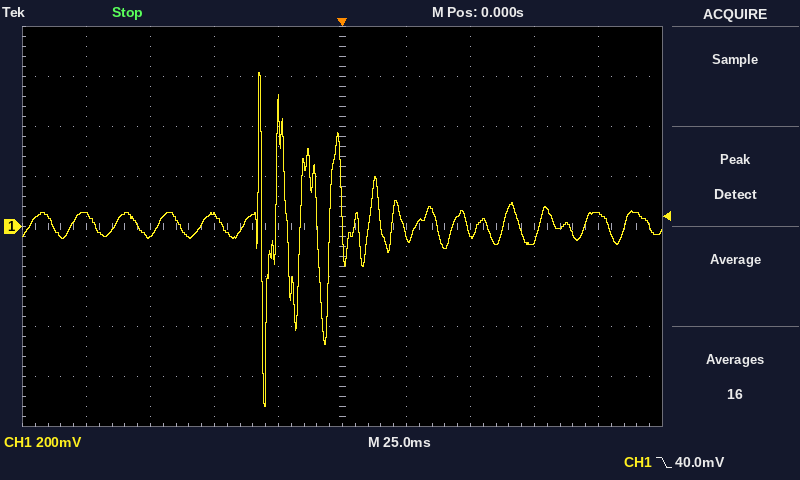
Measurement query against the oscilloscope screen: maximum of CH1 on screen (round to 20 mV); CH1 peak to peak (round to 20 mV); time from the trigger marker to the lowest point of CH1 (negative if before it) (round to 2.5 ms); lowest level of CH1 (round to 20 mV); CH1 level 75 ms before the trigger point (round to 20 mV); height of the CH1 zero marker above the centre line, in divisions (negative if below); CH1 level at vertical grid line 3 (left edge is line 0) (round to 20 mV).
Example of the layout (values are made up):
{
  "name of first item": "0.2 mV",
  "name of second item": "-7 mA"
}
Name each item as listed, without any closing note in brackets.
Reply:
{
  "maximum of CH1 on screen": "620 mV",
  "CH1 peak to peak": "1.34 V",
  "time from the trigger marker to the lowest point of CH1 (negative if before it)": "-30.0 ms",
  "lowest level of CH1": "-720 mV",
  "CH1 level 75 ms before the trigger point": "-40 mV",
  "height of the CH1 zero marker above the centre line, in divisions": "0.0 div",
  "CH1 level at vertical grid line 3 (left edge is line 0)": "40 mV"
}
